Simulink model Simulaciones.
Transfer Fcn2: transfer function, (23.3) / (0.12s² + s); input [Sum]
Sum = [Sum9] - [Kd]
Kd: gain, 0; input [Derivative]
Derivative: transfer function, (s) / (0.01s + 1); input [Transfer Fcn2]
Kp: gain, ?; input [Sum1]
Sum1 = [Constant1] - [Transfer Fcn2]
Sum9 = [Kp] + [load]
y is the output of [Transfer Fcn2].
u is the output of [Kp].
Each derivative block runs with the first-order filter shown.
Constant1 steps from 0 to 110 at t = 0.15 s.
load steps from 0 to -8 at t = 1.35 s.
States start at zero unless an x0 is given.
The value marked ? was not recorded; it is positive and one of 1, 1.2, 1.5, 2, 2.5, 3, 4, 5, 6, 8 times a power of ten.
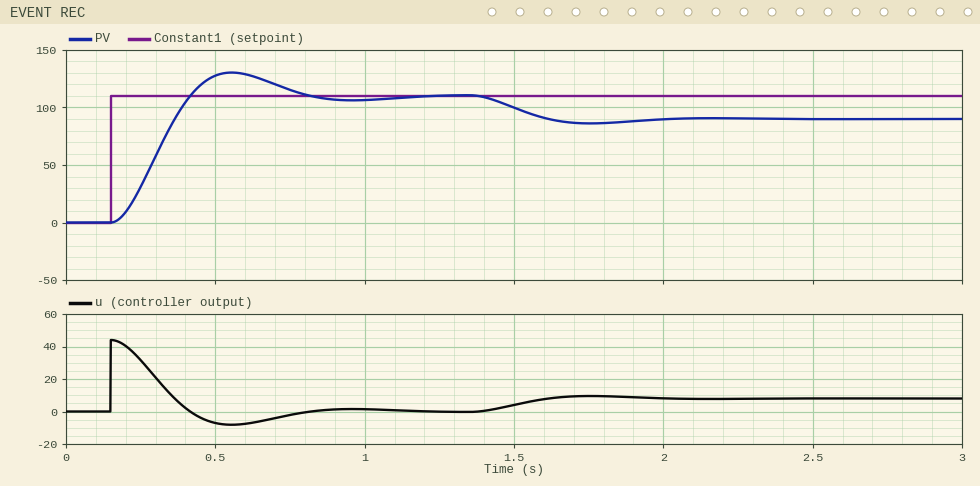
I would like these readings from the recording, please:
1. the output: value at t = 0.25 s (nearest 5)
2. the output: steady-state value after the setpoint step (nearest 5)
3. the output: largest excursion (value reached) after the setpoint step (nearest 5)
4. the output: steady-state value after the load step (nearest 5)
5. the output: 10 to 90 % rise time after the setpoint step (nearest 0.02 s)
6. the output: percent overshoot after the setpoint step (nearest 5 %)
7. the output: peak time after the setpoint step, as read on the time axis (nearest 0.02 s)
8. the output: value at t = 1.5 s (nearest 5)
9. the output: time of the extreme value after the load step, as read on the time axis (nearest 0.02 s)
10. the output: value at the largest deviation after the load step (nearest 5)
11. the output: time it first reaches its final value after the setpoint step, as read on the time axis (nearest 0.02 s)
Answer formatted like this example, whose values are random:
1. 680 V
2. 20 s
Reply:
1. 30
2. 110
3. 130
4. 90
5. 0.18 s
6. 20 %
7. 0.56 s
8. 100
9. 1.76 s
10. 85
11. 0.42 s
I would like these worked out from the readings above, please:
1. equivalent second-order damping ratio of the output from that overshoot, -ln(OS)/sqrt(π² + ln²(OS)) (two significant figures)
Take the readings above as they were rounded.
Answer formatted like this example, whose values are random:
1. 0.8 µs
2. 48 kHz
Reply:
1. 0.46
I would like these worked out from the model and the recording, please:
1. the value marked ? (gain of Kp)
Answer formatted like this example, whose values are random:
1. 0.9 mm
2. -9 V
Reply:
1. 0.4
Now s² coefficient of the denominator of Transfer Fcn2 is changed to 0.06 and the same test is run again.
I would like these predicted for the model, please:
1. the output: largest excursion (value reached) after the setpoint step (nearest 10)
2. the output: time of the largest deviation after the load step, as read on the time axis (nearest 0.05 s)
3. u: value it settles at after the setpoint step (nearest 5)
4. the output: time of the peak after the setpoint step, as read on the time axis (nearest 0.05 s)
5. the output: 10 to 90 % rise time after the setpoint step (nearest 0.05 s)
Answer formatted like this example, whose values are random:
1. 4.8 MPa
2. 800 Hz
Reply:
1. 120
2. 1.70 s
3. 0
4. 0.50 s
5. 0.15 s
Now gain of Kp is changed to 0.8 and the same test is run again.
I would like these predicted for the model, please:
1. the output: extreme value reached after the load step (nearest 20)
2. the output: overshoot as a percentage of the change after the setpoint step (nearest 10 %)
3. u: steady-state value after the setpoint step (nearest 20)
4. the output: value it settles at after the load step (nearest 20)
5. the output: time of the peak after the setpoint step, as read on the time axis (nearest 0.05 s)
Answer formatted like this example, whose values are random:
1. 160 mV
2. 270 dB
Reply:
1. 100
2. 30 %
3. 0
4. 100
5. 0.40 s
